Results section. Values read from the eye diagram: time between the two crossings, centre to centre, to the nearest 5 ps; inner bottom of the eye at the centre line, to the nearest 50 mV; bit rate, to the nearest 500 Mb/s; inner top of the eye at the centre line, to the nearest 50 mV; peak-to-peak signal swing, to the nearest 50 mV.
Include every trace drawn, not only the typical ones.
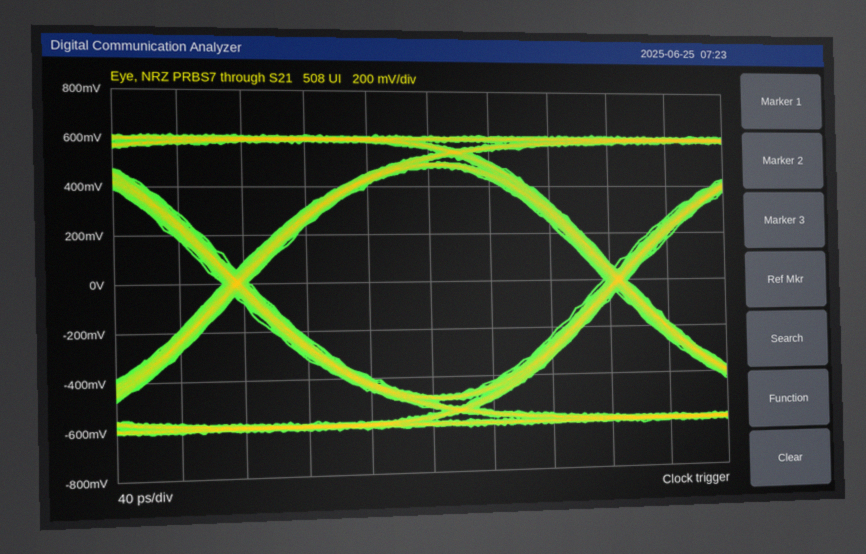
250 ps
-500 mV
4.0 Gb/s
500 mV
1.25 V
